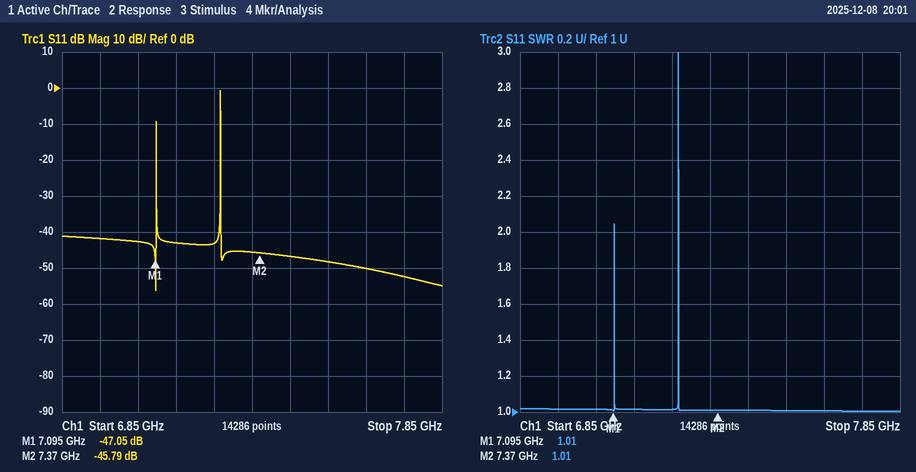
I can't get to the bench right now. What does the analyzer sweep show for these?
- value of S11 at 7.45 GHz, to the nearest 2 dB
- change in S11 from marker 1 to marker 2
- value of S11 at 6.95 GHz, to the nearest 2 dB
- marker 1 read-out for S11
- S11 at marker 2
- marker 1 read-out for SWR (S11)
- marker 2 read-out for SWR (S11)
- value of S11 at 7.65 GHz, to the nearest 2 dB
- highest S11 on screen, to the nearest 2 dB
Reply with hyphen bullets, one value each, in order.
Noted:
- -46 dB
- 1.26 dB
- -42 dB
- -47.05 dB
- -45.79 dB
- 1.01
- 1.01
- -50 dB
- 0 dB
